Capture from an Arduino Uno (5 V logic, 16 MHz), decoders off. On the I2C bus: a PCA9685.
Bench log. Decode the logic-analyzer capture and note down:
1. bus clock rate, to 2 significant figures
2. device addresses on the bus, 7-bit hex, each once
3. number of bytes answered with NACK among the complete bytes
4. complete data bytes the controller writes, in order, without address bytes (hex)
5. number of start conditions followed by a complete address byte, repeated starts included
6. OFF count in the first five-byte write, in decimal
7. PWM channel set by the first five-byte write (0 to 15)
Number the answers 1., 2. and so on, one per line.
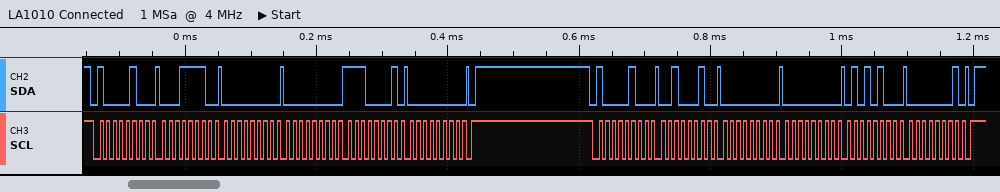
1. 100 kHz
2. 0x42
3. 0
4. 1E 00 00 E1 00 22 00 00 54 01
5. 2
6. 225
7. 6
